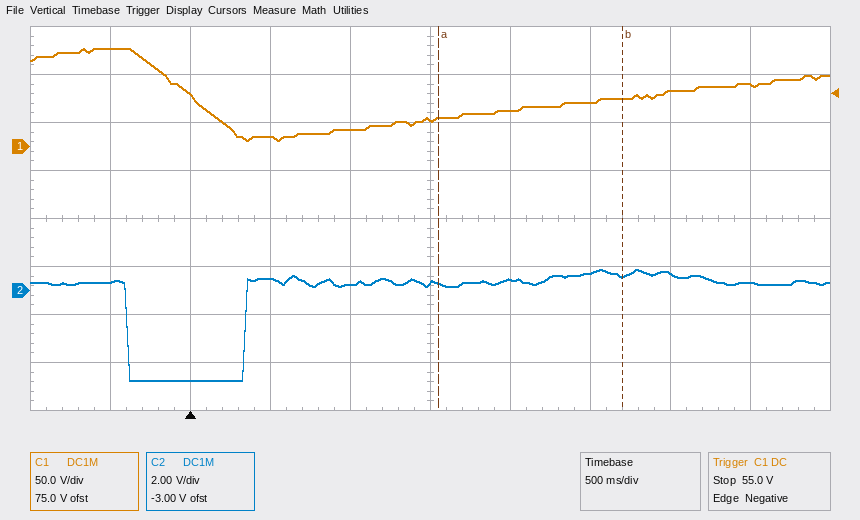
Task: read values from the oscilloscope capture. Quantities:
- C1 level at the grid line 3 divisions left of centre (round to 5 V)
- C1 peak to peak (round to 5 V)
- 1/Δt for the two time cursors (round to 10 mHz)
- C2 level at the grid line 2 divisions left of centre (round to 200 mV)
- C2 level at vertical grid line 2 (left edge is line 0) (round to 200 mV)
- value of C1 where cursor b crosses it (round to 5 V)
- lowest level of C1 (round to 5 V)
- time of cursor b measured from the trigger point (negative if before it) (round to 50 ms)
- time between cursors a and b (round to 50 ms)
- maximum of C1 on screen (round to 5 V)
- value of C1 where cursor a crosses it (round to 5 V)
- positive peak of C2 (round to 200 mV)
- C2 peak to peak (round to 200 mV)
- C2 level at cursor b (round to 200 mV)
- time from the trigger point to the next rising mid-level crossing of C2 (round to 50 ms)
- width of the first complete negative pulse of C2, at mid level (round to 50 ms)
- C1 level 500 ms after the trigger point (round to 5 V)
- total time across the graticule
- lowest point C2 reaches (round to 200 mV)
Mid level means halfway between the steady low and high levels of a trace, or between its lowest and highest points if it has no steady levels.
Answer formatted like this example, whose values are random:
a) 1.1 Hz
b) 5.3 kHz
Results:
a) 55 V
b) 95 V
c) 870 mHz
d) 400 mV
e) -3.8 V
f) 50 V
g) 5 V
h) +2.70 s
i) 1.15 s
j) 100 V
k) 30 V
l) 800 mV
m) 4.6 V
n) 600 mV
o) 350 ms
p) 750 ms
q) 10 V
r) 5 s
s) -3.8 V
